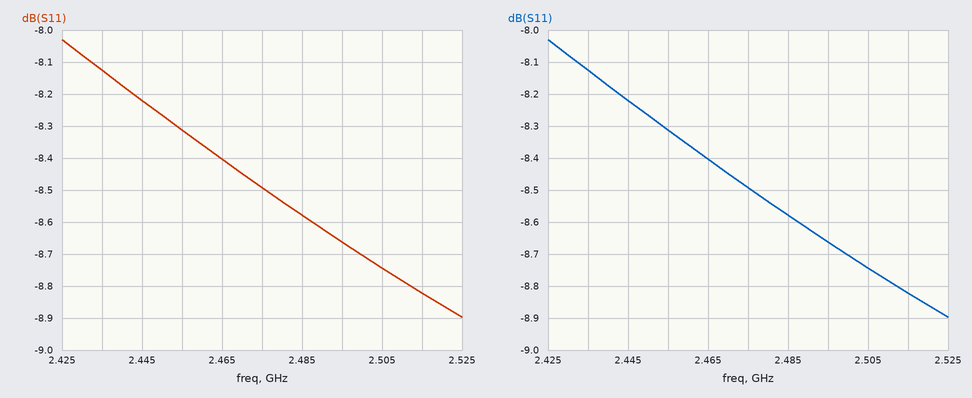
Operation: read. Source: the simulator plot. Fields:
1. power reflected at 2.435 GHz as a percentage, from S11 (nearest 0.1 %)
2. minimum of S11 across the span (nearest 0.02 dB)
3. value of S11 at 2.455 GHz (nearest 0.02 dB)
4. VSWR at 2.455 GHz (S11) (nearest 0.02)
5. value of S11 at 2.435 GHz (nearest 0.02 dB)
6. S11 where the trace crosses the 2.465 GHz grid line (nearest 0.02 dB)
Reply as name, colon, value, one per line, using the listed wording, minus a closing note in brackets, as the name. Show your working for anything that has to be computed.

power reflected at 2.435 GHz as a percentage, from S11: 10^(-8.12/10) ≈ 15.4 %
minimum of S11 across the span: -8.90 dB
value of S11 at 2.455 GHz: -8.32 dB
VSWR at 2.455 GHz (S11): |Γ| = 10^(-8.32/20) = 0.3837; VSWR = (1 + 0.3837)/(1 − 0.3837) ≈ 2.25, so 2.24 to the nearest 0.02
value of S11 at 2.435 GHz: -8.12 dB
S11 where the trace crosses the 2.465 GHz grid line: -8.40 dB
